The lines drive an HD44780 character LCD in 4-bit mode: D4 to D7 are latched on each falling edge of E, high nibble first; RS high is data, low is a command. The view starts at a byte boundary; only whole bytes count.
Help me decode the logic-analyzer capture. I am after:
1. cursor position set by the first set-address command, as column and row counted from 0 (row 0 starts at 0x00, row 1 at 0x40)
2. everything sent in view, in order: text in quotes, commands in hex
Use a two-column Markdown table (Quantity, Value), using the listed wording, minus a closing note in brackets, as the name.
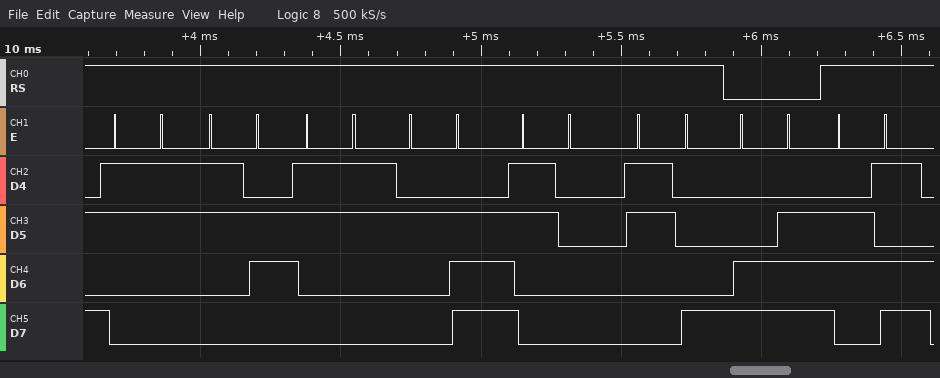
| Quantity | Value |
|---|---|
| cursor position set by the first set-address command, as column and row counted from 0 | column 14, row 1 |
| everything sent in view, in order: text in quotes, commands in hex | "363.08" 0xCE "m" |
